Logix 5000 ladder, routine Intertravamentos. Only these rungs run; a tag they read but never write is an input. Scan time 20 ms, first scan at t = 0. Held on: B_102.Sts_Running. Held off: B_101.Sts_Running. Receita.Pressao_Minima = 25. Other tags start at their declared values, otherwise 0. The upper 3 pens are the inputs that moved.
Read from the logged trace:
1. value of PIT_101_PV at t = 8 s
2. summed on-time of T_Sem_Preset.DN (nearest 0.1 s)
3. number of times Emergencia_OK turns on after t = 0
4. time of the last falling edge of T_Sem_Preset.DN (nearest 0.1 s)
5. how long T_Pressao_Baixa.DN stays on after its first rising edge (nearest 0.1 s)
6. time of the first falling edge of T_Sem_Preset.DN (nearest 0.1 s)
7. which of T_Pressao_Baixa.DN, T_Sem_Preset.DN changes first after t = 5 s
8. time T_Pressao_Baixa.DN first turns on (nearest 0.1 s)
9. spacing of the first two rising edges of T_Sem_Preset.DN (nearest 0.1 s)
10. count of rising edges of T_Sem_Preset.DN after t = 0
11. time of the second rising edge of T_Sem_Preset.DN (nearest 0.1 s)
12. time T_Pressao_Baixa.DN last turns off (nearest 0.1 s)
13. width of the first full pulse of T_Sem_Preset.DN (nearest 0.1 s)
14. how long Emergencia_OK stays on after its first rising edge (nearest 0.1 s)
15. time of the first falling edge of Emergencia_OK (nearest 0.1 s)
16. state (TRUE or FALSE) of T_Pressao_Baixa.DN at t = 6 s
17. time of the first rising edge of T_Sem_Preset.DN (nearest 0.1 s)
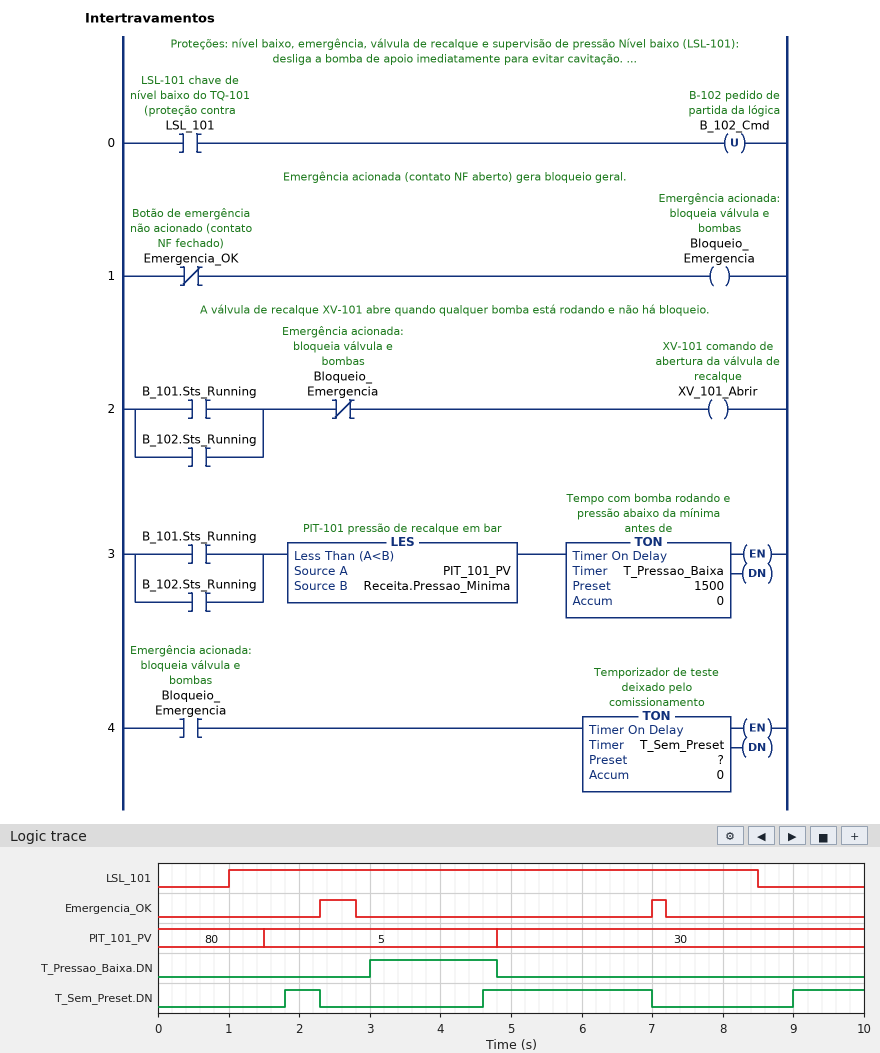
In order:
30
3.9 s
2
7.0 s
1.8 s
2.3 s
T_Sem_Preset.DN
3.0 s
2.8 s
3
4.6 s
4.8 s
0.5 s
0.5 s
2.8 s
FALSE
1.8 s
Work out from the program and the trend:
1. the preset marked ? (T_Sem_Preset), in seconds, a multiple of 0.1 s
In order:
1.8 s
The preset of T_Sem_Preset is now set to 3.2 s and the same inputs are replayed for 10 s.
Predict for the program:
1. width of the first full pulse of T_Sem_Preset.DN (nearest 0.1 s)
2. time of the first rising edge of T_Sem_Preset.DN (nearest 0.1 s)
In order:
1.0 s
6.0 s
